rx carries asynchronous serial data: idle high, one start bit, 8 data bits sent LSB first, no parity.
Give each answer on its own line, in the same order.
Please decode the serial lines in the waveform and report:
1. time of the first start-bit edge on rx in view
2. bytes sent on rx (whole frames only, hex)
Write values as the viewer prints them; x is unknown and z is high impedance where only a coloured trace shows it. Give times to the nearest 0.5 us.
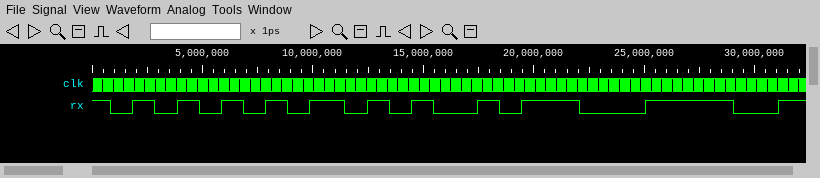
1 us
55, A5, 3C
